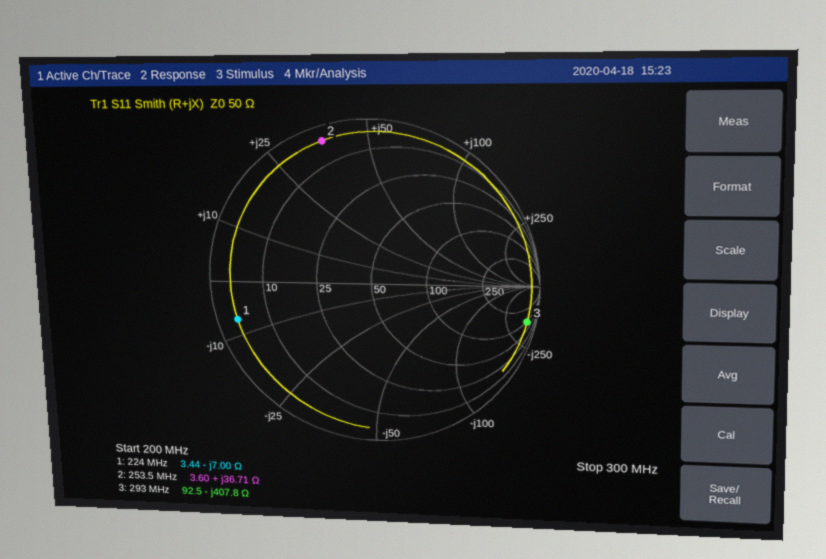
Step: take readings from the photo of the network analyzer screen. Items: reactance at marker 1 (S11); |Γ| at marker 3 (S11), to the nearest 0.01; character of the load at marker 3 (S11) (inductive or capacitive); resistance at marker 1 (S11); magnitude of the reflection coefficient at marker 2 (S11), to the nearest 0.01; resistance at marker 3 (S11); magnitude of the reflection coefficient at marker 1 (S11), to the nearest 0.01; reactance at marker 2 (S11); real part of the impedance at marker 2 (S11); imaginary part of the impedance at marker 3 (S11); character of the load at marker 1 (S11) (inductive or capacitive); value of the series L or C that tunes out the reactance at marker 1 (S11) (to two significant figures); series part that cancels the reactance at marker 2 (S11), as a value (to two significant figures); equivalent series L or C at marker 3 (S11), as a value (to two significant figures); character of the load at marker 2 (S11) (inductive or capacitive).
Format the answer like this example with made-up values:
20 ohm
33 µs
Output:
-7.00 Ω
0.95
capacitive
3.44 Ω
0.91
92.5 Ω
0.87
+36.71 Ω
3.60 Ω
-407.8 Ω
capacitive
5.0 nH
17 pF
1.3 pF
inductive
